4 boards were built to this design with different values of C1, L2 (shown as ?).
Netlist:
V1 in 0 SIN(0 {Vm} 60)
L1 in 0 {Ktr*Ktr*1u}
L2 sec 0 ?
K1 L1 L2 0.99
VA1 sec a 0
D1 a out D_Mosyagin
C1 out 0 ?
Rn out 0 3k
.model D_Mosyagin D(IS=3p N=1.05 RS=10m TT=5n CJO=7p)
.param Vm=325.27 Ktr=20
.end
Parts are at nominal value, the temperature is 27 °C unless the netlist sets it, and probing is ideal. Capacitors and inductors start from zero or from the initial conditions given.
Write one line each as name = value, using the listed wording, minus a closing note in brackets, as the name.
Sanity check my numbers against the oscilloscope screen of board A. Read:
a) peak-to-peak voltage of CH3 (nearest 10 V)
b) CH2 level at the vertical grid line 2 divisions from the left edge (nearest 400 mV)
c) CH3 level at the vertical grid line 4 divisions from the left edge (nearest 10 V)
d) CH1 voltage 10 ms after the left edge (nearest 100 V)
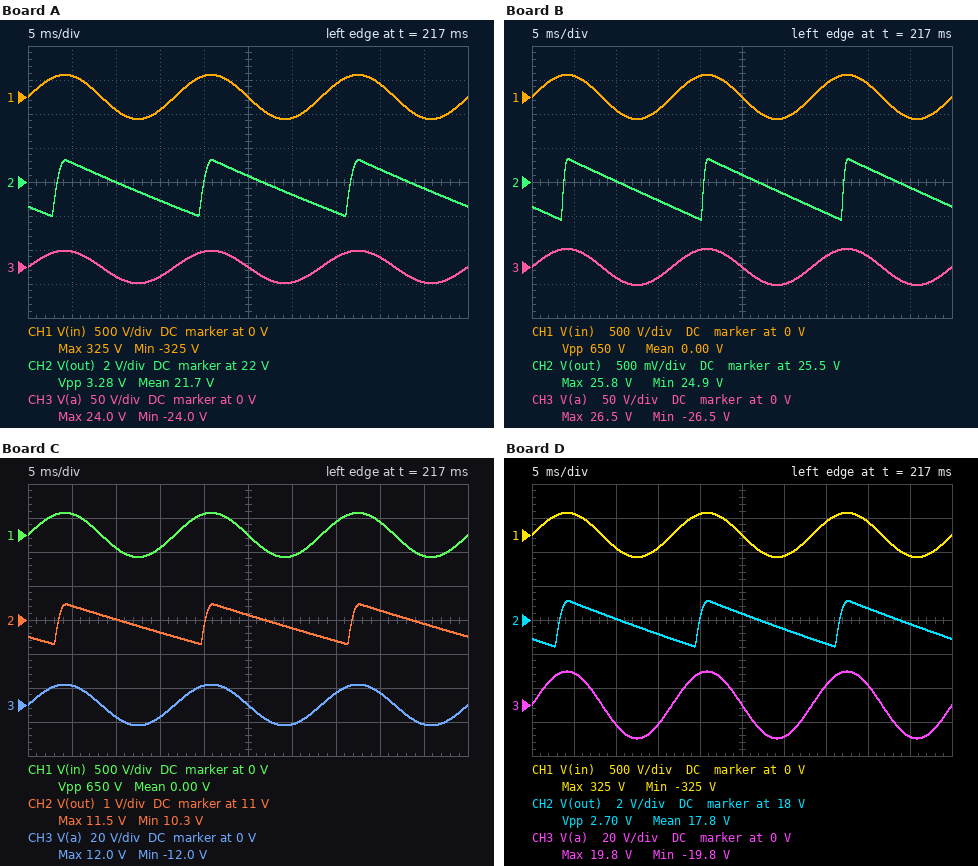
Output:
peak-to-peak voltage of CH3 = 50 V
CH2 level at the vertical grid line 2 divisions from the left edge = 22.0 V
CH3 level at the vertical grid line 4 divisions from the left edge = 20 V
CH1 voltage 10 ms after the left edge = -200 V
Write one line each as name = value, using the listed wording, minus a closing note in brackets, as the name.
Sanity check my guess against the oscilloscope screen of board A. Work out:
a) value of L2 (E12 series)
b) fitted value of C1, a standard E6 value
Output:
value of L2 = 2.2 µH
fitted value of C1, a standard E6 value = 33 µF
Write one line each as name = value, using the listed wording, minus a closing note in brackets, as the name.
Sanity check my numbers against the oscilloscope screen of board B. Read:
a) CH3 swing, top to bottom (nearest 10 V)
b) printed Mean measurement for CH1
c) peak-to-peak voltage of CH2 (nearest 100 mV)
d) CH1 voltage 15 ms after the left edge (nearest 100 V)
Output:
CH3 swing, top to bottom = 50 V
printed Mean measurement for CH1 = 0.00 V
peak-to-peak voltage of CH2 = 900 mV
CH1 voltage 15 ms after the left edge = -200 V
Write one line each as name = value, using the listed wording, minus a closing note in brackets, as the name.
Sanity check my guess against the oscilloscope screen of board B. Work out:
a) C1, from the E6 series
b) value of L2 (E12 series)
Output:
C1, from the E6 series = 150 µF
value of L2 = 2.7 µH
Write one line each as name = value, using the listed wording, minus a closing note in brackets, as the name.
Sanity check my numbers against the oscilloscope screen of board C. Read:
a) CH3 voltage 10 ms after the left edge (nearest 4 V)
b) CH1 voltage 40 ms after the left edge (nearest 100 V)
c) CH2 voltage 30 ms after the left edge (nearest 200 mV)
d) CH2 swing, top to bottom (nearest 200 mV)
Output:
CH3 voltage 10 ms after the left edge = -8 V
CH1 voltage 40 ms after the left edge = 200 V
CH2 voltage 30 ms after the left edge = 10.8 V
CH2 swing, top to bottom = 1.2 V
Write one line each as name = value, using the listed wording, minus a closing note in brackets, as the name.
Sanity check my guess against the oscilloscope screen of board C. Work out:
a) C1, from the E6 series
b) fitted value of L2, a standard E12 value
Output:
C1, from the E6 series = 47 µF
fitted value of L2, a standard E12 value = 560 nH
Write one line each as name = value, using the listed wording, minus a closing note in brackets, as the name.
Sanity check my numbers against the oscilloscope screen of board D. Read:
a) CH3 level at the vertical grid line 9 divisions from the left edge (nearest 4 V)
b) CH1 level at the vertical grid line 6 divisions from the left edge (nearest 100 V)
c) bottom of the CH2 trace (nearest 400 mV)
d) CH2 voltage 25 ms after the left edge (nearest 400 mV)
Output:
CH3 level at the vertical grid line 9 divisions from the left edge = -20 V
CH1 level at the vertical grid line 6 divisions from the left edge = -300 V
bottom of the CH2 trace = 16.4 V
CH2 voltage 25 ms after the left edge = 18.4 V
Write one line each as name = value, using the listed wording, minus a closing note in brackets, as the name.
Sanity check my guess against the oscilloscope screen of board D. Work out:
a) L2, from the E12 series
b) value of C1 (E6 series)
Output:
L2, from the E12 series = 1.5 µH
value of C1 = 33 µF
